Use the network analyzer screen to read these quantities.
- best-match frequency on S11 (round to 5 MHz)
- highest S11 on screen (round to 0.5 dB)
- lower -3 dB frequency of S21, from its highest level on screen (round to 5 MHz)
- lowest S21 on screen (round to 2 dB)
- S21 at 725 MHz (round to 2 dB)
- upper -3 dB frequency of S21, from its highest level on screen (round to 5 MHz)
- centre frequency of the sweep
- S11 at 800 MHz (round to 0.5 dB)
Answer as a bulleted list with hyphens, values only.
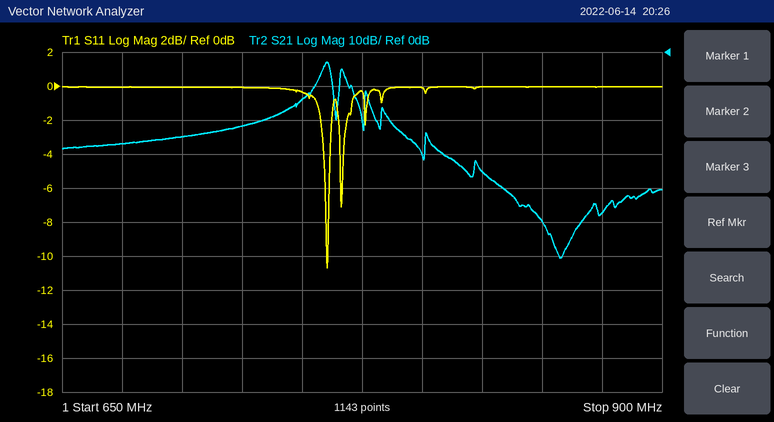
- 760 MHz
- 0.0 dB
- 760 MHz
- -60 dB
- -22 dB
- 760 MHz
- 775 MHz
- 0.0 dB
